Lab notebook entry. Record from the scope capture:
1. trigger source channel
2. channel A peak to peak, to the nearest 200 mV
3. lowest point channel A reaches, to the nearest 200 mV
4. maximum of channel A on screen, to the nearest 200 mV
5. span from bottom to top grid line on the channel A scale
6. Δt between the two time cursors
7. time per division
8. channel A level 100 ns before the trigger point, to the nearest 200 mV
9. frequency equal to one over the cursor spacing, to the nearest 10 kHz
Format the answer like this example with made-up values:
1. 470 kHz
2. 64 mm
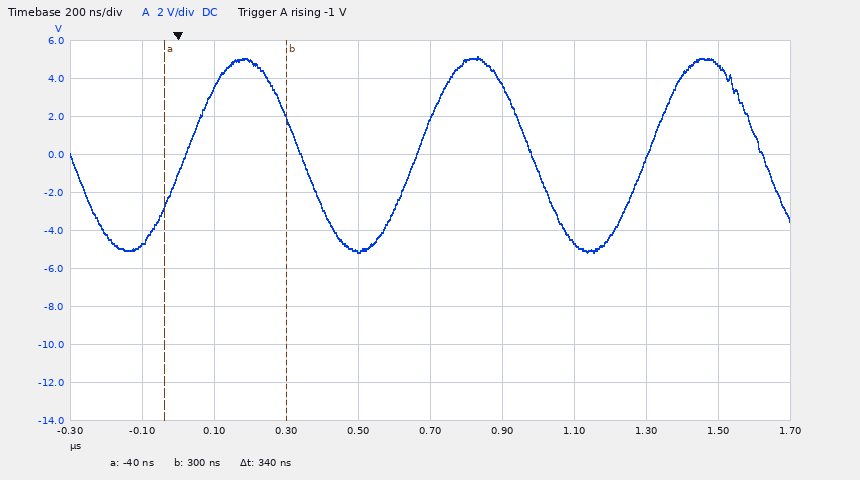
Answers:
1. channel A
2. 10.4 V
3. -5.2 V
4. 5.2 V
5. 20 V
6. 340 ns
7. 200 ns
8. -4.8 V
9. 2.94 MHz
